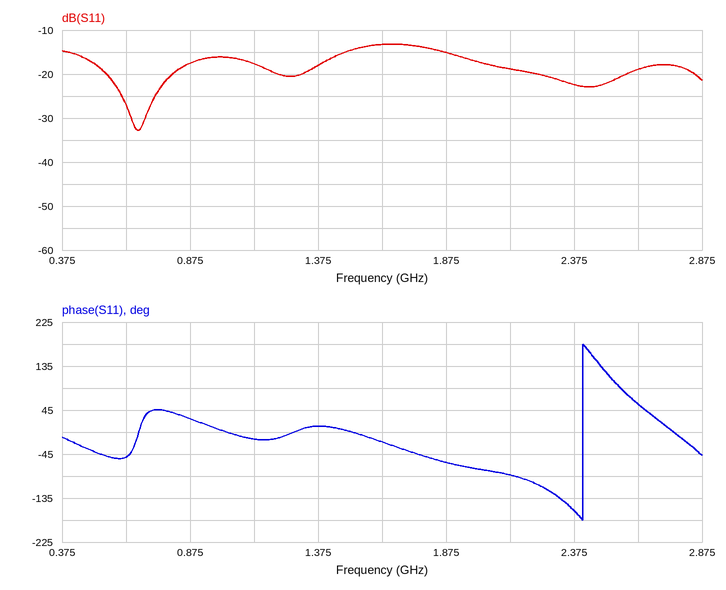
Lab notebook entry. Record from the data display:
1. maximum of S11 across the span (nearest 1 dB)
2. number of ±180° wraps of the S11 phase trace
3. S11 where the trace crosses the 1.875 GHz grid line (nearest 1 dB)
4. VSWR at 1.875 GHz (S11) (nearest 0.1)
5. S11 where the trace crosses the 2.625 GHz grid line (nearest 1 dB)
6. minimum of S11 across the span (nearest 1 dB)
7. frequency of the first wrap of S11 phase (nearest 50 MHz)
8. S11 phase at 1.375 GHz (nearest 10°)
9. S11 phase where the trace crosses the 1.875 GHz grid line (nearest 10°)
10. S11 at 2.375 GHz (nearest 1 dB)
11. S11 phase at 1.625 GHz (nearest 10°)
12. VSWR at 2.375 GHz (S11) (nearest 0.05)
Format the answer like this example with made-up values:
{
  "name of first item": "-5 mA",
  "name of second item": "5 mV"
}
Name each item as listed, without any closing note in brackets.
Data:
{
  "maximum of S11 across the span": "-13 dB",
  "number of ±180° wraps of the S11 phase trace": "1",
  "S11 where the trace crosses the 1.875 GHz grid line": "-15 dB",
  "VSWR at 1.875 GHz (S11)": "1.4",
  "S11 where the trace crosses the 2.625 GHz grid line": "-19 dB",
  "minimum of S11 across the span": "-33 dB",
  "frequency of the first wrap of S11 phase": "2.40 GHz",
  "S11 phase at 1.375 GHz": "10°",
  "S11 phase where the trace crosses the 1.875 GHz grid line": "-60°",
  "S11 at 2.375 GHz": "-22 dB",
  "S11 phase at 1.625 GHz": "-20°",
  "VSWR at 2.375 GHz (S11)": "1.15"
}
